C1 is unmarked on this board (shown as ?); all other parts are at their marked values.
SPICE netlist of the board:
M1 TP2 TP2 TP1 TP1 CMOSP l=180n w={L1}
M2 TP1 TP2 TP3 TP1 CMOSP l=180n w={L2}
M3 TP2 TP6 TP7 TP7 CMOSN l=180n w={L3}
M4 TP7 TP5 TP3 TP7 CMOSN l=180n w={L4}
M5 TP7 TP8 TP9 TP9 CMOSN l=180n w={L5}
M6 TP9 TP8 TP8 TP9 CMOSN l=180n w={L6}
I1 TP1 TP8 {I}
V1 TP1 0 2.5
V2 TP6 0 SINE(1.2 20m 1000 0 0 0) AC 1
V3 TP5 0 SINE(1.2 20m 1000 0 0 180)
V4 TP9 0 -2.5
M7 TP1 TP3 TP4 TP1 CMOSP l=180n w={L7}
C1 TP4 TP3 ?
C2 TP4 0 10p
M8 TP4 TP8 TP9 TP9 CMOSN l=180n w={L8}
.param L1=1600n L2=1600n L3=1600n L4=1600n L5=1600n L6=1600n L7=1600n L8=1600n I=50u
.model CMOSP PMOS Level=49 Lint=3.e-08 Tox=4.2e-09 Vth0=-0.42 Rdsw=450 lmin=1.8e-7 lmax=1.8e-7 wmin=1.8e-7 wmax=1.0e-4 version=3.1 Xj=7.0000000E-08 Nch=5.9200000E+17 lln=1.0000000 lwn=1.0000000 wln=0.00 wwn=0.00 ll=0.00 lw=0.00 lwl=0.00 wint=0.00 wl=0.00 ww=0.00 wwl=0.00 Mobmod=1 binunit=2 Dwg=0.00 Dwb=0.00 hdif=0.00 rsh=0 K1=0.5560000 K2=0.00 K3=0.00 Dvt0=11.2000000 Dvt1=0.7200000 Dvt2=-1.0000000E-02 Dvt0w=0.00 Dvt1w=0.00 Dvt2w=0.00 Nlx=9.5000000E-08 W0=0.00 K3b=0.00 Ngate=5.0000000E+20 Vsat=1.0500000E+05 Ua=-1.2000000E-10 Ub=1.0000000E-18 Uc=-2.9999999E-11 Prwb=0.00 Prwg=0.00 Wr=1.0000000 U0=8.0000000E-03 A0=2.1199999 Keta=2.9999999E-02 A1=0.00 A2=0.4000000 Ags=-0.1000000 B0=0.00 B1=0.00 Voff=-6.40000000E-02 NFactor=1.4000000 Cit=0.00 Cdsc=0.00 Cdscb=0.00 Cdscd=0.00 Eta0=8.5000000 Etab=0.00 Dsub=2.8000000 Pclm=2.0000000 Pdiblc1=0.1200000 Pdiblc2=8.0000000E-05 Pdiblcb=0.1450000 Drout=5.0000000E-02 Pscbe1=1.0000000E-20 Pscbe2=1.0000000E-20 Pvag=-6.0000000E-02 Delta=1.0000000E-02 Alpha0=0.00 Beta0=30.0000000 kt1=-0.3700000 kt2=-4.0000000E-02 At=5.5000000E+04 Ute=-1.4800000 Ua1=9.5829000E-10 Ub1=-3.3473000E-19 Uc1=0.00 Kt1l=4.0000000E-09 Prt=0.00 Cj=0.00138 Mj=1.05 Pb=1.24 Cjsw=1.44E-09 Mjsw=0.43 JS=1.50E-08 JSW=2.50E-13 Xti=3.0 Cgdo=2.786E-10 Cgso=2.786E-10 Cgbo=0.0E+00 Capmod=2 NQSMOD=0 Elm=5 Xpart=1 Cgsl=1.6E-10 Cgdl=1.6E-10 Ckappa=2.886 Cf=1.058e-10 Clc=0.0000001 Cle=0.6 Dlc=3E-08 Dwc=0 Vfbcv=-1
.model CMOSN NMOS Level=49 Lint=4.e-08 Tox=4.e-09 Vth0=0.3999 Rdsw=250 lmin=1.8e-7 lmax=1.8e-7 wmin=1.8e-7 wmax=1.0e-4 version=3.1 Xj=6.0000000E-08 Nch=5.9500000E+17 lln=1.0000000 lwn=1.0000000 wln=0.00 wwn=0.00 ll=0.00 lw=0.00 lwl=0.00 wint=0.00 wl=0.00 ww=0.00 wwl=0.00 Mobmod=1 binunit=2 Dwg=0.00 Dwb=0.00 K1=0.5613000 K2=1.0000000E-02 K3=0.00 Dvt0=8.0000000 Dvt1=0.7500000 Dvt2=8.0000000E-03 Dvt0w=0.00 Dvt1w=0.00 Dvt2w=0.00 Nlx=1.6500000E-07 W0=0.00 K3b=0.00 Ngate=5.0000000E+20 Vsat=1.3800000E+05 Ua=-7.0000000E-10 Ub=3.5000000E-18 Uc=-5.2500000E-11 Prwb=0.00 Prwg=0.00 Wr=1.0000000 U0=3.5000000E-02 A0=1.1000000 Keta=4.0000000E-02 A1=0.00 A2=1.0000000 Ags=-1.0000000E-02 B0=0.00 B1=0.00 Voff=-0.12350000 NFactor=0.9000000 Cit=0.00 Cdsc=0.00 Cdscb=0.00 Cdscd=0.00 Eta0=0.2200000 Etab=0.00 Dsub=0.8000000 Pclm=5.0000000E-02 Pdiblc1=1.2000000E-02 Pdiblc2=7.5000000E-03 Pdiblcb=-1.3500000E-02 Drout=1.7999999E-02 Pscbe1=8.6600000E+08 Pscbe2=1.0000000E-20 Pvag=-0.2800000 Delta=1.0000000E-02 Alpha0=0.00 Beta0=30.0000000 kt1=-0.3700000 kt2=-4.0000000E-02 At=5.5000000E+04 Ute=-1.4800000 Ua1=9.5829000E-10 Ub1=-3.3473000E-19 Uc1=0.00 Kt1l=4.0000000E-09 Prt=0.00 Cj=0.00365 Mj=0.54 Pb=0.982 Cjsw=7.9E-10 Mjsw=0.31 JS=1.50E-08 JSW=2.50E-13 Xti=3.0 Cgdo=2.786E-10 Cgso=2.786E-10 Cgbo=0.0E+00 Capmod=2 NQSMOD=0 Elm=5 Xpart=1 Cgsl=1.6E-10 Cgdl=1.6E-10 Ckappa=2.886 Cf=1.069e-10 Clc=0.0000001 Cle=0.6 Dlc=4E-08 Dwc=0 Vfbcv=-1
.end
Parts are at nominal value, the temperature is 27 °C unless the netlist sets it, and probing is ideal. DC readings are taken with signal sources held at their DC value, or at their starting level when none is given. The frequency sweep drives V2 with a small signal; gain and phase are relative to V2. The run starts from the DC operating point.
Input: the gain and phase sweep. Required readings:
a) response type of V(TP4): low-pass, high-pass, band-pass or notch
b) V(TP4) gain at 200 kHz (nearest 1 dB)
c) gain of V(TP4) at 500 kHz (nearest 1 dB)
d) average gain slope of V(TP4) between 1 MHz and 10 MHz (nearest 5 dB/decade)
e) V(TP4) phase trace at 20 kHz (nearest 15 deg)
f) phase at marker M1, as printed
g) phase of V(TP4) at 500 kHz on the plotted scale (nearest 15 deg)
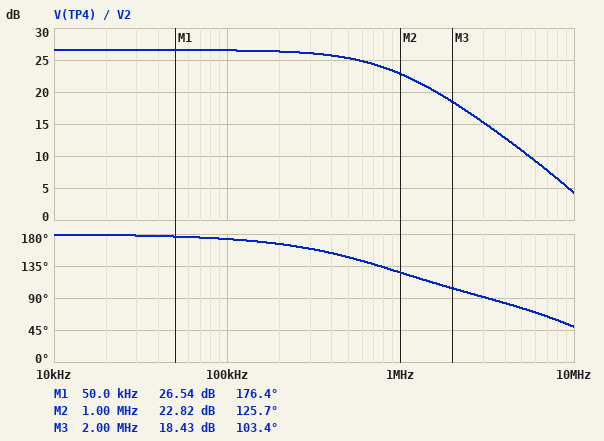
low-pass
26 dB
25 dB
-20 dB/decade
180 deg
176.4 deg
150 deg
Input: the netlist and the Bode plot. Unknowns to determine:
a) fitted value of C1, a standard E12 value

1.8 pF
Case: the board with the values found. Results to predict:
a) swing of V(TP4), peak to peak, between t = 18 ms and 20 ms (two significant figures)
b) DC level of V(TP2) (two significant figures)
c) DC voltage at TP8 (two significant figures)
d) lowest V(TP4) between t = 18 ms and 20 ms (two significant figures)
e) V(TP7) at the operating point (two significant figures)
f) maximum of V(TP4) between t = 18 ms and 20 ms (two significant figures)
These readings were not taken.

1.8 V
1.7 V
-1.9 V
-870 mV
600 mV
900 mV
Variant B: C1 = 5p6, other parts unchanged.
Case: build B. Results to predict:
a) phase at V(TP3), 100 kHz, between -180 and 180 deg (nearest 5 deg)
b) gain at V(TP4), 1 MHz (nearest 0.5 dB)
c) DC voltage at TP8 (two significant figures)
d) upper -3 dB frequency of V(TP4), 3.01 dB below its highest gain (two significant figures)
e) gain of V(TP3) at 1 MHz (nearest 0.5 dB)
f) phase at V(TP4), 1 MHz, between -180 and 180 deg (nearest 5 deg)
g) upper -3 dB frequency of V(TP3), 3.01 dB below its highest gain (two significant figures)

-10 deg
18.0 dB
-1.9 V
390 kHz
9.0 dB
100 deg
450 kHz
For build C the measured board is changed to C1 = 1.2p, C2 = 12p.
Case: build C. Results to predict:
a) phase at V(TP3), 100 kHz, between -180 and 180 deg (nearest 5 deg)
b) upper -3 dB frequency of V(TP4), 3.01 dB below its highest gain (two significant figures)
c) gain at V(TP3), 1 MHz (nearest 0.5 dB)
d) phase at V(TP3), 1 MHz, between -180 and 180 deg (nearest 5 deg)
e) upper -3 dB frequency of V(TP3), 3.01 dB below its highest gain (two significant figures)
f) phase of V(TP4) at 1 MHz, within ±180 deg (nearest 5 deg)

0 deg
940 kHz
14.0 dB
-15 deg
3.5 MHz
130 deg
